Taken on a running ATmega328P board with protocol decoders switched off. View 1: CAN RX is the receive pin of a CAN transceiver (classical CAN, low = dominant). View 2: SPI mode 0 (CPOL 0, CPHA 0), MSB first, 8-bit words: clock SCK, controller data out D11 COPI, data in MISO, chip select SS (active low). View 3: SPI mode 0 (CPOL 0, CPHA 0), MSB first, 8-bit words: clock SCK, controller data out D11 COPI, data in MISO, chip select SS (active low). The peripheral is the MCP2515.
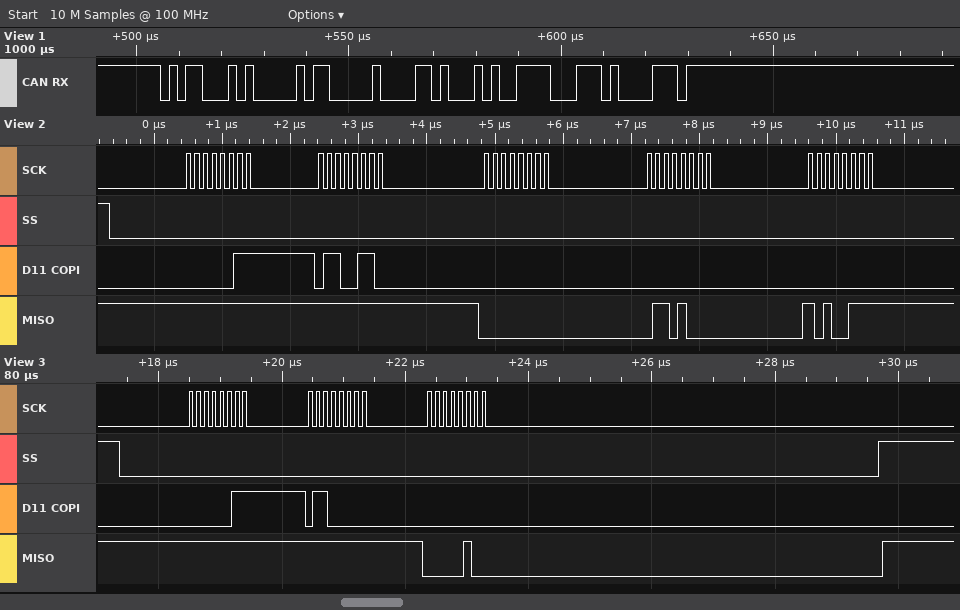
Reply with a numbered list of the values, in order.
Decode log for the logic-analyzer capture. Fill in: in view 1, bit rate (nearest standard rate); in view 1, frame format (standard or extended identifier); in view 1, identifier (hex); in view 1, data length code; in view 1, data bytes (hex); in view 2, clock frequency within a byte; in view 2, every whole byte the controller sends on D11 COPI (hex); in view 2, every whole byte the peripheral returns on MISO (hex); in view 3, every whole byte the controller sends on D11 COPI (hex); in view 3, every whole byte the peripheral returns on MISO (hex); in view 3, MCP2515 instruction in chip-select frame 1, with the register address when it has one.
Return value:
1. 500 kbit/s
2. standard
3. 0x58A
4. 3
5. 00 68 A7
6. 8 MHz
7. 0x03 0x66 0x00 0x00 0x00
8. 0xFF 0xFF 0x00 0x68 0xA7
9. 03 60 00
10. FF FF 04
11. READ 0x60
